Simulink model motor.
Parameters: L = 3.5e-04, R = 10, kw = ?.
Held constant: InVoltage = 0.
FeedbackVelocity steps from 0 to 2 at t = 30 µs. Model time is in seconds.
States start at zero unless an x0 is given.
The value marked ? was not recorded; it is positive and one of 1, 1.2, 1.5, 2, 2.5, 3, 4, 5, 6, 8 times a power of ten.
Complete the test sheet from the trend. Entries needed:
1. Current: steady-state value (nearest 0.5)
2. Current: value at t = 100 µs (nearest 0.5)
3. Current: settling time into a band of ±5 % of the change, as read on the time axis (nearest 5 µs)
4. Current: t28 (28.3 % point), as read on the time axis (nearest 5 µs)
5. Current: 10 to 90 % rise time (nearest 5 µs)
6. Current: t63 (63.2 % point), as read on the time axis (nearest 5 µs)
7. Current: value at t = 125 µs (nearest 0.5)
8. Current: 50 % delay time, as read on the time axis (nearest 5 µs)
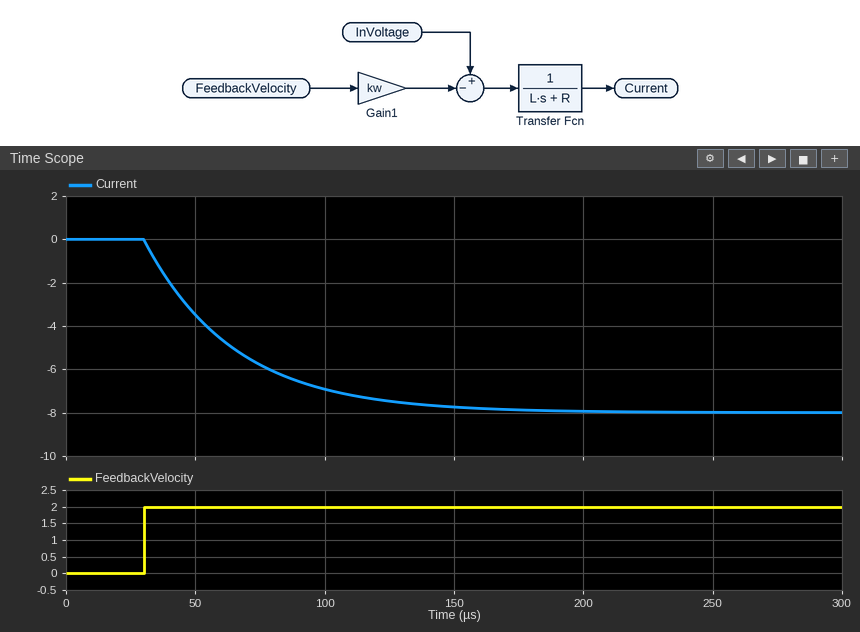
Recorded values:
-8.0
-7.0
135 µs
40 µs
75 µs
65 µs
-7.5
55 µs
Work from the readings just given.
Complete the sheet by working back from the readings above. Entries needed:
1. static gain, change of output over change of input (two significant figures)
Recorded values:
-4.0
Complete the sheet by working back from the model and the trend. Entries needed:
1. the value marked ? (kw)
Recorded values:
40
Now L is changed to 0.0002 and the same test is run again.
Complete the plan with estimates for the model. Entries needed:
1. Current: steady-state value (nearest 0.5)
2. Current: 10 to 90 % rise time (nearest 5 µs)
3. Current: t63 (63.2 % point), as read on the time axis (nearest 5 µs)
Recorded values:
-8.0
45 µs
50 µs
